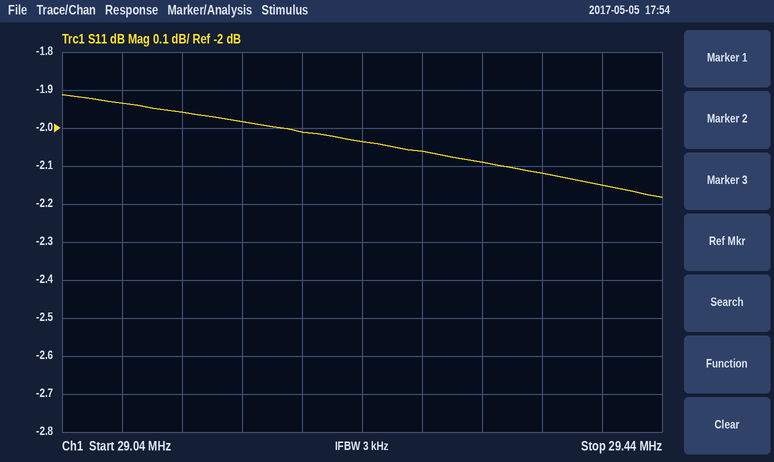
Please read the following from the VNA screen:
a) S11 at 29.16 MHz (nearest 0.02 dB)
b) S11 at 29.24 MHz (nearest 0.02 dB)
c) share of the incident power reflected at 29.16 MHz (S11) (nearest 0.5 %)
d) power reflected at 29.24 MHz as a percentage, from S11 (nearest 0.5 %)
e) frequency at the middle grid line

-1.98 dB
-2.04 dB
63.5 %
62.5 %
29.24 MHz
